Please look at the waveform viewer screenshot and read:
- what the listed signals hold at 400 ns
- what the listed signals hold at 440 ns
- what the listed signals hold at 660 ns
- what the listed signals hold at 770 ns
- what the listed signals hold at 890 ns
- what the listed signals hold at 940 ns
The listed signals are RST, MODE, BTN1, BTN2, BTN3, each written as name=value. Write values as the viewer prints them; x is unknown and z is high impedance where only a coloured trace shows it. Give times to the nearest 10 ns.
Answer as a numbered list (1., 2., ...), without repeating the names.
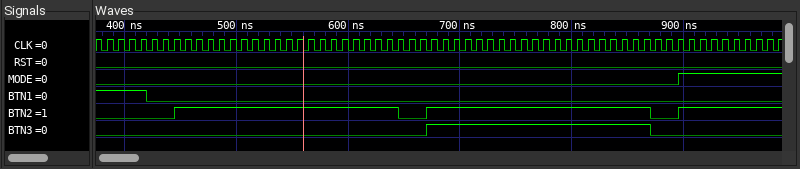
1. RST=0, MODE=0, BTN1=1, BTN2=0, BTN3=0
2. RST=0, MODE=0, BTN1=0, BTN2=0, BTN3=0
3. RST=0, MODE=0, BTN1=0, BTN2=0, BTN3=0
4. RST=0, MODE=0, BTN1=0, BTN2=1, BTN3=1
5. RST=0, MODE=0, BTN1=0, BTN2=0, BTN3=0
6. RST=0, MODE=1, BTN1=0, BTN2=1, BTN3=0
